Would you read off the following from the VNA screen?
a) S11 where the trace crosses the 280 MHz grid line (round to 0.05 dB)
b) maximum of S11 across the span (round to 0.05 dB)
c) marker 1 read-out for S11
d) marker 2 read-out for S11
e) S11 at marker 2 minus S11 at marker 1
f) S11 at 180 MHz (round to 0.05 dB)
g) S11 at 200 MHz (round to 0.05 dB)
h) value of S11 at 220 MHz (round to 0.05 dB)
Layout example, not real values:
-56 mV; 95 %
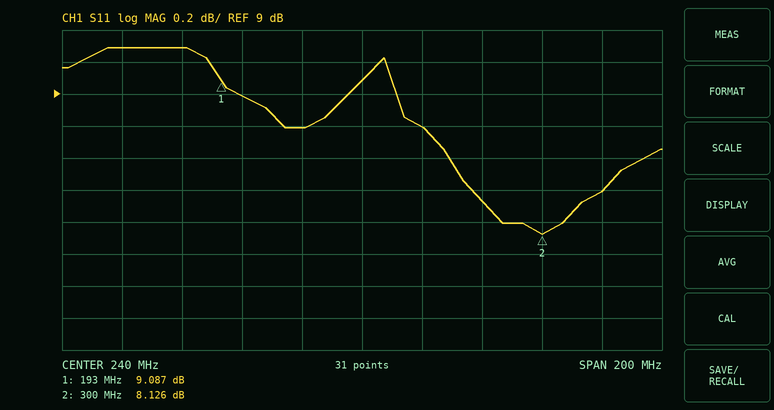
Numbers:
8.35 dB; 9.30 dB; 9.087 dB; 8.126 dB; -0.961 dB; 9.30 dB; 9.00 dB; 8.80 dB
